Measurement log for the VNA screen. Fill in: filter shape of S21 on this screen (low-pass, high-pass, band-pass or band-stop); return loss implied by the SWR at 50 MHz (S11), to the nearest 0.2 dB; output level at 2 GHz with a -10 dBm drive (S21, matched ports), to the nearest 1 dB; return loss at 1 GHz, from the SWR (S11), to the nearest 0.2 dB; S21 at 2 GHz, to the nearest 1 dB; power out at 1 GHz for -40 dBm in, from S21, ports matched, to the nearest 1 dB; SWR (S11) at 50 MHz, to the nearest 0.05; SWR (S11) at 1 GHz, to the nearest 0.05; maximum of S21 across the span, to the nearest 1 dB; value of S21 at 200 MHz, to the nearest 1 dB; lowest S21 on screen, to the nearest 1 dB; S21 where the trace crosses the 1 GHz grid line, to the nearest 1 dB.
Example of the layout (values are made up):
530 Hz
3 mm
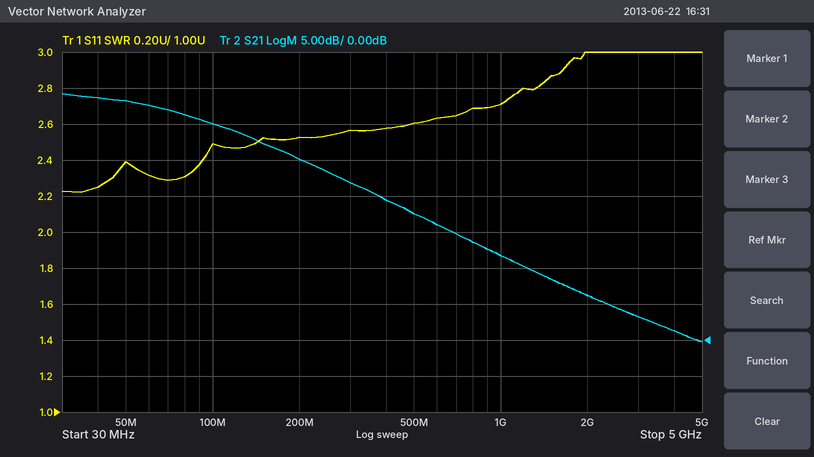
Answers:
low-pass
7.8 dB
-4 dBm
6.8 dB
6 dB
-28 dBm
2.40
2.70
34 dB
25 dB
0 dB
12 dB
